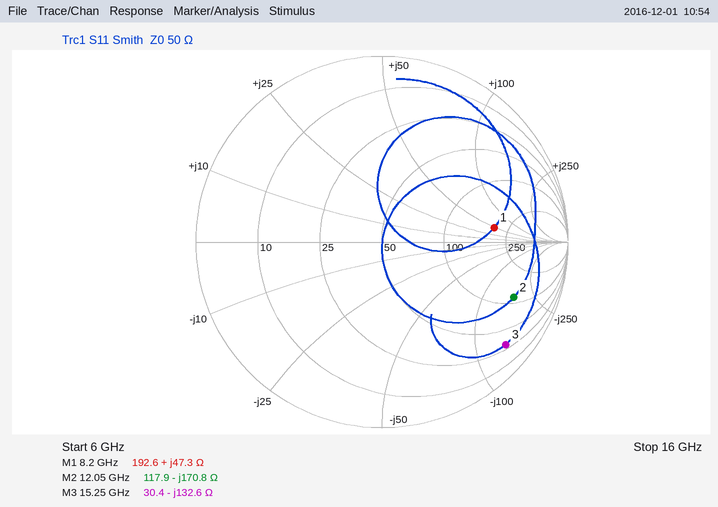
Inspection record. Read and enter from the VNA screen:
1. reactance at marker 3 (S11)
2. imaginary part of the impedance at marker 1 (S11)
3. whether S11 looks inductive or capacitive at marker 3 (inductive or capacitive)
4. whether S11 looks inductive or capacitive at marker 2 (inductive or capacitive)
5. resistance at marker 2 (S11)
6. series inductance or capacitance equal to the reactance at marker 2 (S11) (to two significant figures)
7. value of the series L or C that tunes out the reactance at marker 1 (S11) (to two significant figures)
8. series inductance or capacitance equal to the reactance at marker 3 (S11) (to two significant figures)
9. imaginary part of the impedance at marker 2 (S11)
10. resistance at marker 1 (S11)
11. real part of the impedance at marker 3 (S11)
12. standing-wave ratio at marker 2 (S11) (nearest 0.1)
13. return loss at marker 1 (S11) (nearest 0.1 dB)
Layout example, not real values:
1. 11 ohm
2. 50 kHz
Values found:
1. -132.6 Ω
2. +47.3 Ω
3. capacitive
4. capacitive
5. 117.9 Ω
6. 77 fF
7. 410 fF
8. 79 fF
9. -170.8 Ω
10. 192.6 Ω
11. 30.4 Ω
12. 7.6
13. 4.3 dB
